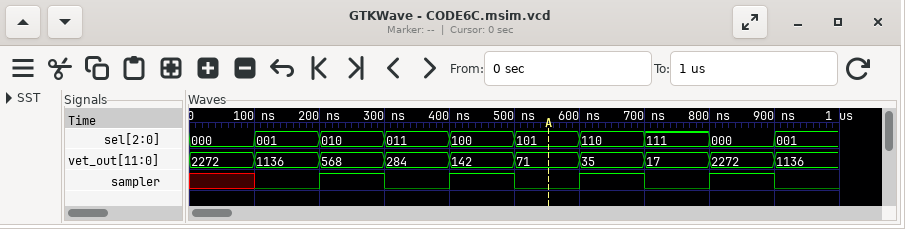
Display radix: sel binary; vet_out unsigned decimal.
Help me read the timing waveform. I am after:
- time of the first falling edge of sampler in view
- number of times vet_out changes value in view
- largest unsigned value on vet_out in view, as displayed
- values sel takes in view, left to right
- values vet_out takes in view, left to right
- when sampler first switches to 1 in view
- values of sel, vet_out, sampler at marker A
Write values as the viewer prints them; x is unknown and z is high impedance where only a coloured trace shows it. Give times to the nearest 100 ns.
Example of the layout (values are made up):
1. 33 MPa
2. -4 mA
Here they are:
1. 300 ns
2. 9
3. 2272
4. 000, 001, 010, 011, 100, 101, 110, 111, 000, 001
5. 2272, 1136, 568, 284, 142, 71, 35, 17, 2272, 1136
6. 200 ns
7. sel=101, vet_out=71, sampler=0
